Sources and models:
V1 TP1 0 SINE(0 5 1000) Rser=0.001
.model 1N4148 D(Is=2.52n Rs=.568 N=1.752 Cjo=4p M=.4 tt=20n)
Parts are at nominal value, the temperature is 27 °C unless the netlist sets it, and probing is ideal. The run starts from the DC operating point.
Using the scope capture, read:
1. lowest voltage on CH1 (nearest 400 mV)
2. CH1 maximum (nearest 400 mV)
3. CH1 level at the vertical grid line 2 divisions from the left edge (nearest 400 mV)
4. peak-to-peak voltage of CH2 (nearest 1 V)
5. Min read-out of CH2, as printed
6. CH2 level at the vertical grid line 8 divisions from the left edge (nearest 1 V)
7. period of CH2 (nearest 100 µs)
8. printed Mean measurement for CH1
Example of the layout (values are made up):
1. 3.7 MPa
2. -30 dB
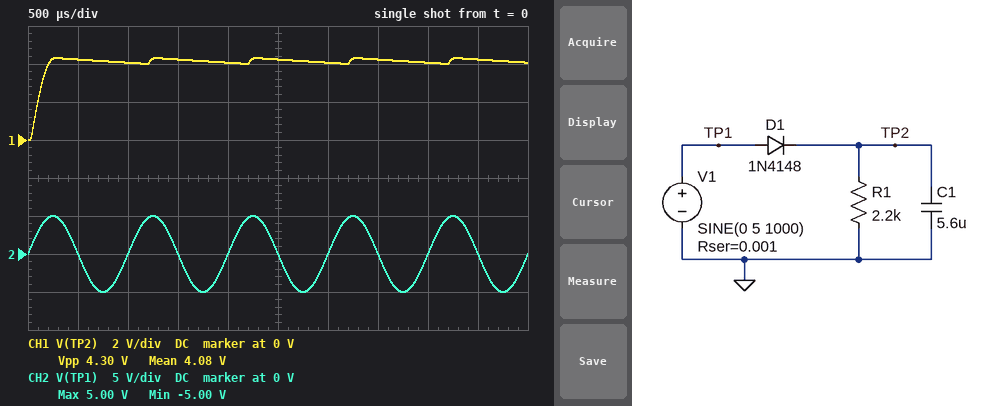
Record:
1. 0 V
2. 4.4 V
3. 4.0 V
4. 10 V
5. -5.00 V
6. 0 V
7. 1.0 ms
8. 4.08 V
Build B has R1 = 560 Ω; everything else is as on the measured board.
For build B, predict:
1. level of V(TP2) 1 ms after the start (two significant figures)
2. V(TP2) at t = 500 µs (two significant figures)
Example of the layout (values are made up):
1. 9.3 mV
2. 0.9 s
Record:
1. 3.4 V
2. 4.0 V
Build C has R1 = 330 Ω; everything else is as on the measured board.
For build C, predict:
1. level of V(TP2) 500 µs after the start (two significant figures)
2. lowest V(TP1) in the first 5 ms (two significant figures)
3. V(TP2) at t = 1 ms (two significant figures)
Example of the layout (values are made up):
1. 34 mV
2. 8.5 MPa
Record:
1. 3.8 V
2. -5.0 V
3. 2.9 V
